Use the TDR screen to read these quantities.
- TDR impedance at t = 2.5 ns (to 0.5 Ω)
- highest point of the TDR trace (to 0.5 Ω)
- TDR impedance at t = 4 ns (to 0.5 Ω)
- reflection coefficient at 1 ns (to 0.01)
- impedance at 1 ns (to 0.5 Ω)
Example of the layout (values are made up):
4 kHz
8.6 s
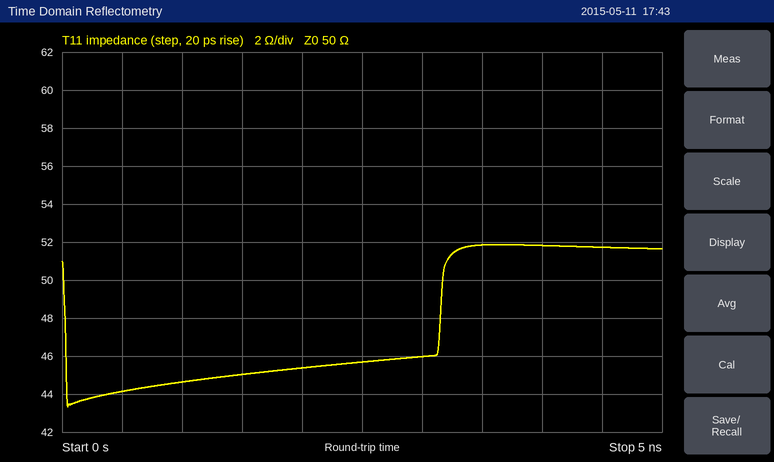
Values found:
45.5 Ω
52.0 Ω
52.0 Ω
-0.06
44.5 Ω
